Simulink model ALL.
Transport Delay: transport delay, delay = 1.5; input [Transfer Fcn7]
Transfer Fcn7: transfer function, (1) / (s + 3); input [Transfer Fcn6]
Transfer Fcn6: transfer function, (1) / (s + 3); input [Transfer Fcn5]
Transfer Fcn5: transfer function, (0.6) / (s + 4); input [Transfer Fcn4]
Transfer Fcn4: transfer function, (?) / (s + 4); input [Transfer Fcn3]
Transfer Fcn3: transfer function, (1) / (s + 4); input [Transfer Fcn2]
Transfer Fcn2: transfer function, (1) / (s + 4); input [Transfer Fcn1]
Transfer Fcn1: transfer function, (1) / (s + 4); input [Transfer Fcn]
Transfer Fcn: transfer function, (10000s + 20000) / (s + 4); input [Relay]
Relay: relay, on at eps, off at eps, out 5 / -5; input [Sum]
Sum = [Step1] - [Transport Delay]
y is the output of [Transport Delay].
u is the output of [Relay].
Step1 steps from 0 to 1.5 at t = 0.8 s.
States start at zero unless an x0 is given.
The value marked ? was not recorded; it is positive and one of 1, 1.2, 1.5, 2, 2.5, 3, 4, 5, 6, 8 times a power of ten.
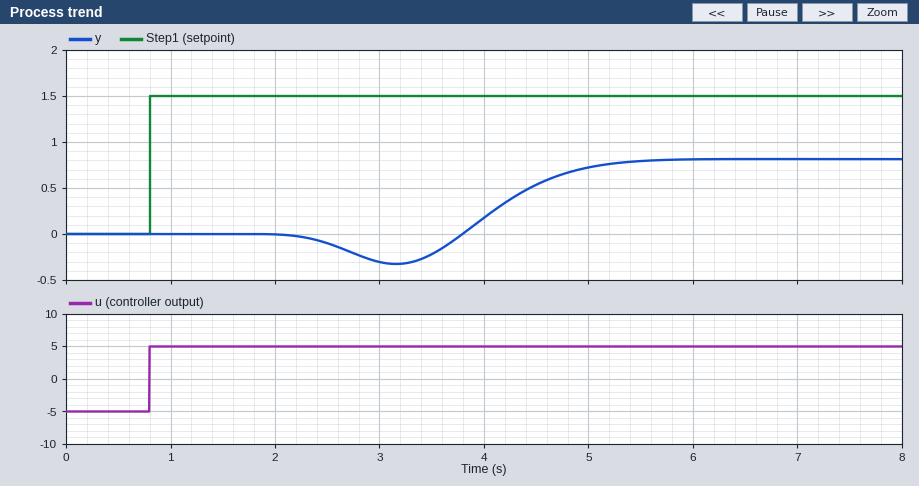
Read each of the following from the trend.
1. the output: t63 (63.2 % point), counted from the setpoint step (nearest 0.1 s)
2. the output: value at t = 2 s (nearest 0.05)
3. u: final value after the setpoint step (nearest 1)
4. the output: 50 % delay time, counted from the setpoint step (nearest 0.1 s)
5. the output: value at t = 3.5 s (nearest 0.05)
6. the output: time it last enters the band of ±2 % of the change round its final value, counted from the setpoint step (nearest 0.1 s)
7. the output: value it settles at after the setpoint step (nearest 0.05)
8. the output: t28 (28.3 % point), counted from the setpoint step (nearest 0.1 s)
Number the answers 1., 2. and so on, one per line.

1. 3.7 s
2. 0.00
3. 5
4. 3.5 s
5. -0.20
6. 4.8 s
7. 0.80
8. 3.3 s
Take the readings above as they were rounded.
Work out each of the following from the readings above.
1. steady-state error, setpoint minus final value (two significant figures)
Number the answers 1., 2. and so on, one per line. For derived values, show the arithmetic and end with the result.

1. 1.5 - 0.8 = 0.70
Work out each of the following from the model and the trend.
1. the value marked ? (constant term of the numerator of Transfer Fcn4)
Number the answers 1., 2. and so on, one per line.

1. 0.5
